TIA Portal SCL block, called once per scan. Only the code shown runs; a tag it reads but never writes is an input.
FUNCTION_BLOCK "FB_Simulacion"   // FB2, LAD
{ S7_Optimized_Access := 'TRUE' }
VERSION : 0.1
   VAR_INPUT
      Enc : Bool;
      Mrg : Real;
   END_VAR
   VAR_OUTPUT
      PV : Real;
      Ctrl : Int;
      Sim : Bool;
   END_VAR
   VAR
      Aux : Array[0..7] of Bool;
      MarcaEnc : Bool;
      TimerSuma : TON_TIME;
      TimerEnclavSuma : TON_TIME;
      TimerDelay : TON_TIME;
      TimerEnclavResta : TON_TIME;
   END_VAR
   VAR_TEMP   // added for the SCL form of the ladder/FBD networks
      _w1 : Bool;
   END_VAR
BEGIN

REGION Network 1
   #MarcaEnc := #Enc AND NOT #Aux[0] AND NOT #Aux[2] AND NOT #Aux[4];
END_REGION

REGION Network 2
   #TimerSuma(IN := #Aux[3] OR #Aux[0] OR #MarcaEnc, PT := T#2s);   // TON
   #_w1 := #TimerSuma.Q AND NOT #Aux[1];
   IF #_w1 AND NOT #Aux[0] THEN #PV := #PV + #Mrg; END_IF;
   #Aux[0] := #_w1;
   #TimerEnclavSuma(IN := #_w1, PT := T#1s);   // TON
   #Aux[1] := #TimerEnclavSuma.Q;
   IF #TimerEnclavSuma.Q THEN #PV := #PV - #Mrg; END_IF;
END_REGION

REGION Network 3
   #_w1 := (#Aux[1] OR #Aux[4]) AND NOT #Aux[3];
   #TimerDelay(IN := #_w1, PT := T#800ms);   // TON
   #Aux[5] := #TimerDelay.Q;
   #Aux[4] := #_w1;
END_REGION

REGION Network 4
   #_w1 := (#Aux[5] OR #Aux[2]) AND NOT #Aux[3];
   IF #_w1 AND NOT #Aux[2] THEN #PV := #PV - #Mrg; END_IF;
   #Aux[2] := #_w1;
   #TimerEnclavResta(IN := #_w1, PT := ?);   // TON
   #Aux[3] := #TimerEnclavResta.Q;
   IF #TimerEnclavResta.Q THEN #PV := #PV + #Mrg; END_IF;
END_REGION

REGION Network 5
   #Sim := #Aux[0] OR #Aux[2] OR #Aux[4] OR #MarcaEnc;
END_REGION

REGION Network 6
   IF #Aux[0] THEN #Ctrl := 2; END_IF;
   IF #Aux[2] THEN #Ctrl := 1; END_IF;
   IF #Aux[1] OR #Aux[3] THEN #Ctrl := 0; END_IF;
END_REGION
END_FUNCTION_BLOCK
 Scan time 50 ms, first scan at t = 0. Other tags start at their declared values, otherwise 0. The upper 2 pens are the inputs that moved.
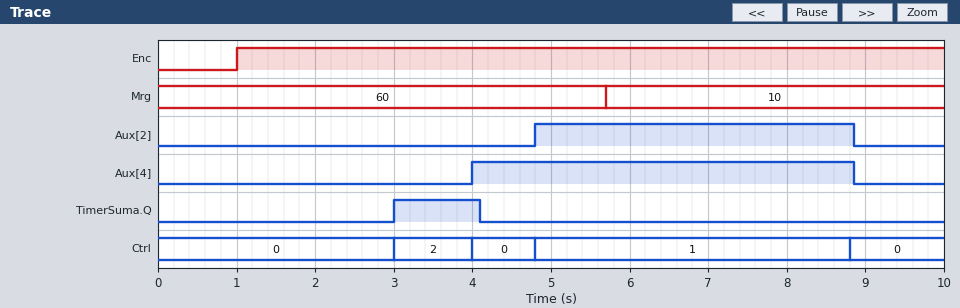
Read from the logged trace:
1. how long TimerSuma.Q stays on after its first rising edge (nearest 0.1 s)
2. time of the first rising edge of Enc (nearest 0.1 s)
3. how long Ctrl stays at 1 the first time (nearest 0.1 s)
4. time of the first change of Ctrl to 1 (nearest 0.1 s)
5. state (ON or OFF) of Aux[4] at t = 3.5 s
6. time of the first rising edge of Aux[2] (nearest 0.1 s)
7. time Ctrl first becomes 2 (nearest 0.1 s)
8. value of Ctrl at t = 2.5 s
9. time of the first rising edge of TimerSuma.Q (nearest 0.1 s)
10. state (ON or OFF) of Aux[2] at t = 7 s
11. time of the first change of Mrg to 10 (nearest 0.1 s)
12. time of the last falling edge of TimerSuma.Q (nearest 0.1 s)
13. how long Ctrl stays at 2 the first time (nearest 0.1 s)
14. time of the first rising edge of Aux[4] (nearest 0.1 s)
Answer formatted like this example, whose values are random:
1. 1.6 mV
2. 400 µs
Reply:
1. 1.1 s
2. 1.0 s
3. 4.0 s
4. 4.8 s
5. OFF
6. 4.8 s
7. 3.0 s
8. 0
9. 3.0 s
10. ON
11. 5.7 s
12. 4.1 s
13. 1.0 s
14. 4.0 s
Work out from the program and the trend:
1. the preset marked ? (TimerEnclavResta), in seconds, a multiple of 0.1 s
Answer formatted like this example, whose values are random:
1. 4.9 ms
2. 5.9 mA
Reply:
1. 4.0 s
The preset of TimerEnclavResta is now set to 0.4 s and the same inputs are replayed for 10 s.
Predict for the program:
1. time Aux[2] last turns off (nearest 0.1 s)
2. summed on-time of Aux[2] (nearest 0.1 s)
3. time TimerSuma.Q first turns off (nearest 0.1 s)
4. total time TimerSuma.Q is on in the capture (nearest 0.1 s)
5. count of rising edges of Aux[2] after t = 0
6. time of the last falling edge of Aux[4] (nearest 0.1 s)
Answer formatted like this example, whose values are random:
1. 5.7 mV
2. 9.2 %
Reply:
1. 9.5 s
2. 0.9 s
3. 4.1 s
4. 2.2 s
5. 2
6. 9.5 s
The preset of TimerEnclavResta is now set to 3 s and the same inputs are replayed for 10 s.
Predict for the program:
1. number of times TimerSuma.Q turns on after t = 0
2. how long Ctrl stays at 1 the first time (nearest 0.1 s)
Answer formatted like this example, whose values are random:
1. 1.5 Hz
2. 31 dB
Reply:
1. 2
2. 3.0 s
